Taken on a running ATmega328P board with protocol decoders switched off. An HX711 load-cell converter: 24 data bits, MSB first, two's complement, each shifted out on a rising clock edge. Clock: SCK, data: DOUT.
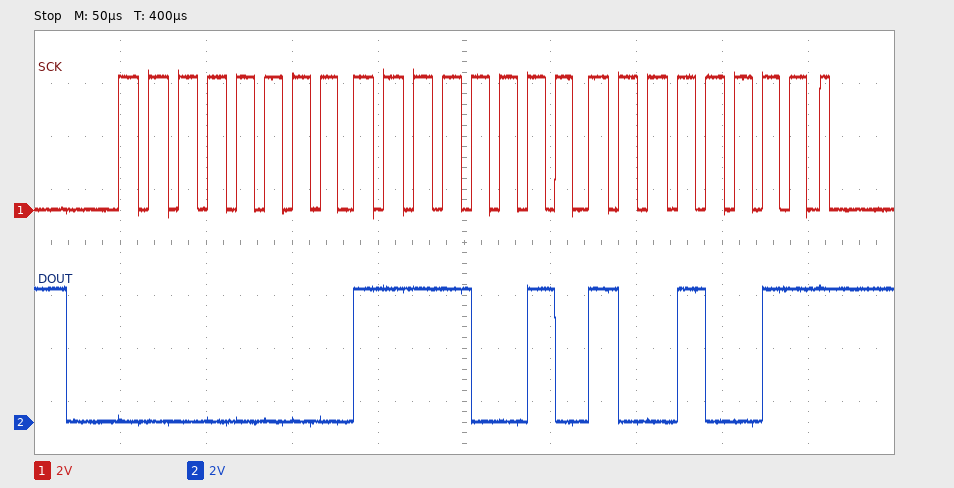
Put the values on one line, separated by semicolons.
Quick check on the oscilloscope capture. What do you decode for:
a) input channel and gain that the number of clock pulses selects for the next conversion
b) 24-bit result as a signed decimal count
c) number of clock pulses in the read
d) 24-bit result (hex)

channel A, gain 128; 62099; 25; 0x00F293
